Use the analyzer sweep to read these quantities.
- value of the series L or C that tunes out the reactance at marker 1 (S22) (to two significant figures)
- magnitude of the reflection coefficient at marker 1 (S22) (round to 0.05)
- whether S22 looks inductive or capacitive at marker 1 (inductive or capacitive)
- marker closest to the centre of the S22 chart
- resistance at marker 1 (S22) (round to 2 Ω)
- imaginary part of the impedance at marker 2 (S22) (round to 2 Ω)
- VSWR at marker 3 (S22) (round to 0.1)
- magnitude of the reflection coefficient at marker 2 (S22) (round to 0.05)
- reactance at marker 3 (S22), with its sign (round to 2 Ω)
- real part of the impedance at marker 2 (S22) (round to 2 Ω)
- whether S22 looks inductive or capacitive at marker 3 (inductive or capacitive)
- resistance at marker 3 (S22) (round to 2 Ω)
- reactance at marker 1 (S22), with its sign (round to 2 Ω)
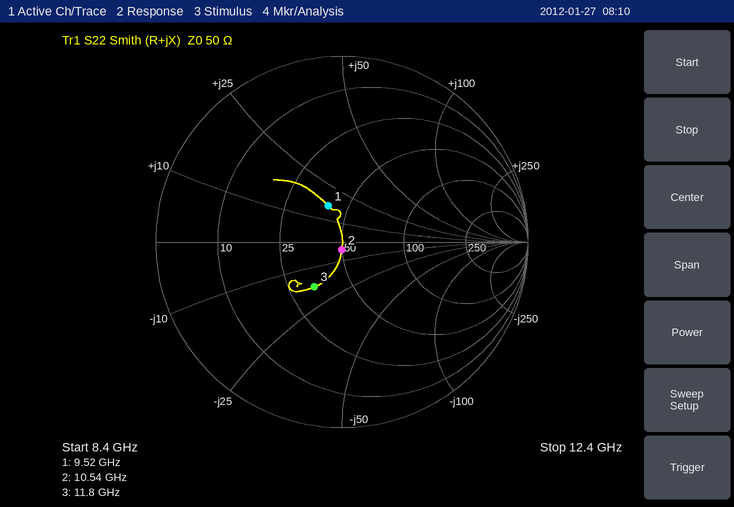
1.0 pF
0.20
inductive
marker 2
40 Ω
-4 Ω
1.8
0.05
-18 Ω
50 Ω
capacitive
34 Ω
+16 Ω
